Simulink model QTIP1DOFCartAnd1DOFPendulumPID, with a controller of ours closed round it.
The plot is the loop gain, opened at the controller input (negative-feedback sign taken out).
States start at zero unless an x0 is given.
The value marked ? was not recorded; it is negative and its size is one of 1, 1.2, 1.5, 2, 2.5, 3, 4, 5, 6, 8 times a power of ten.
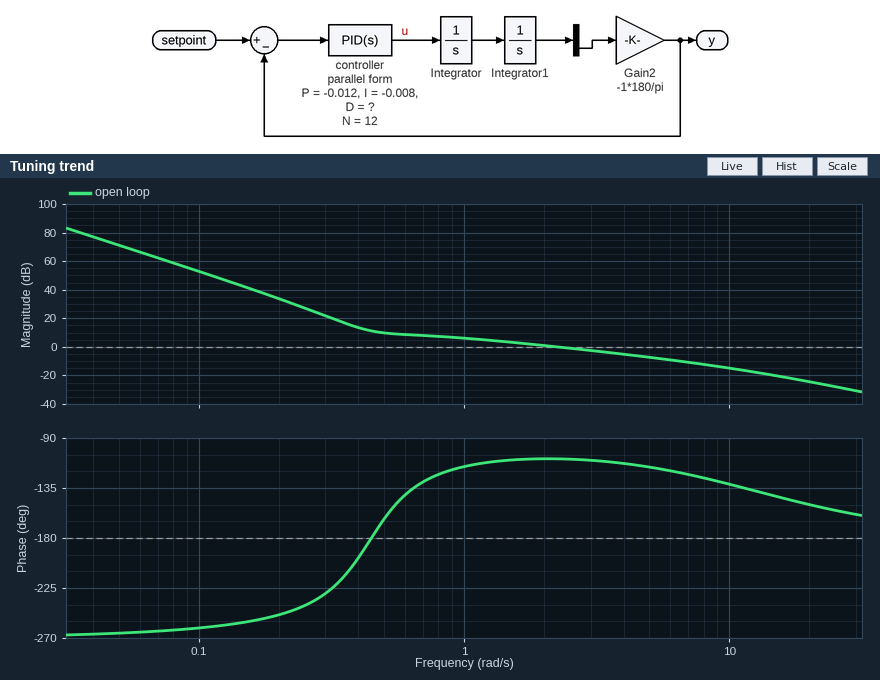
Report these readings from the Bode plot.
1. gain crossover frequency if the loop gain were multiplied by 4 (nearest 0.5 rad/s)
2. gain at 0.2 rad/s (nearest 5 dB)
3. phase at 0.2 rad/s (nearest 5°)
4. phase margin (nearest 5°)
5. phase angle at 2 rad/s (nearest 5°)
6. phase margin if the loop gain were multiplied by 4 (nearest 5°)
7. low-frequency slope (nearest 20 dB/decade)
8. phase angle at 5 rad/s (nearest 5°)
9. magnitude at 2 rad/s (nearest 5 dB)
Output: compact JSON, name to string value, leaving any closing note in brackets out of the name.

{"gain crossover frequency if the loop gain were multiplied by 4": "8.0 rad/s", "gain at 0.2 rad/s": "35 dB", "phase at 0.2 rad/s": "-250°", "phase margin": "70°", "phase angle at 2 rad/s": "-110°", "phase margin if the loop gain were multiplied by 4": "55°", "low-frequency slope": "-60 dB/decade", "phase angle at 5 rad/s": "-115°", "magnitude at 2 rad/s": "0 dB"}
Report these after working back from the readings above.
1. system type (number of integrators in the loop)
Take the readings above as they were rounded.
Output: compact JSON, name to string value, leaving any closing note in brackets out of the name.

{"system type": "3"}
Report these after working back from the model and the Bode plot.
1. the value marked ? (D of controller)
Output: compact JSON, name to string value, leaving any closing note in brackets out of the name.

{"the value marked ?": "-0.04"}
